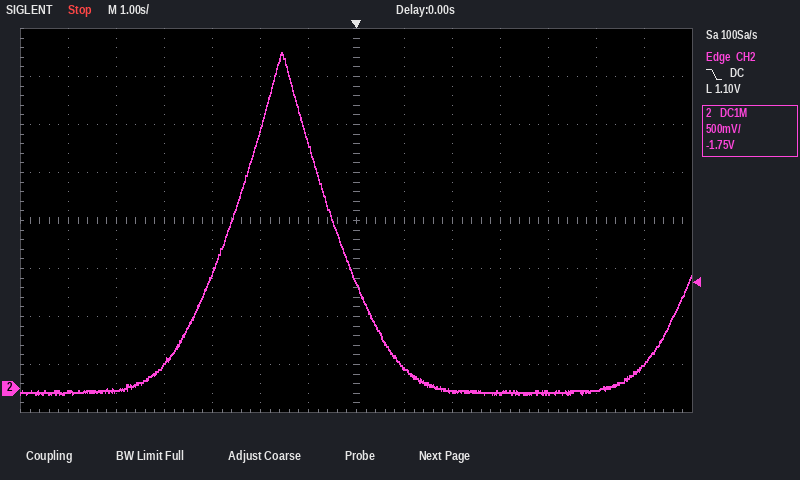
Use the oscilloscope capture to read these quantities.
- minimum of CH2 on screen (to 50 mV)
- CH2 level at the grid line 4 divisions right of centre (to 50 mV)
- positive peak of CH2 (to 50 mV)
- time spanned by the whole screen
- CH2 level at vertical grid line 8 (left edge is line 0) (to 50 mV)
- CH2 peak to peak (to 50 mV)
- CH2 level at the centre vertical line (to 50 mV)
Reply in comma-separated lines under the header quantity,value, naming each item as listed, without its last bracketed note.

quantity,value
minimum of CH2 on screen,-50 mV
CH2 level at the grid line 4 divisions right of centre,-50 mV
positive peak of CH2,3.50 V
time spanned by the whole screen,14 s
CH2 level at vertical grid line 8 (left edge is line 0),200 mV
CH2 peak to peak,3.55 V
CH2 level at the centre vertical line,1.10 V
